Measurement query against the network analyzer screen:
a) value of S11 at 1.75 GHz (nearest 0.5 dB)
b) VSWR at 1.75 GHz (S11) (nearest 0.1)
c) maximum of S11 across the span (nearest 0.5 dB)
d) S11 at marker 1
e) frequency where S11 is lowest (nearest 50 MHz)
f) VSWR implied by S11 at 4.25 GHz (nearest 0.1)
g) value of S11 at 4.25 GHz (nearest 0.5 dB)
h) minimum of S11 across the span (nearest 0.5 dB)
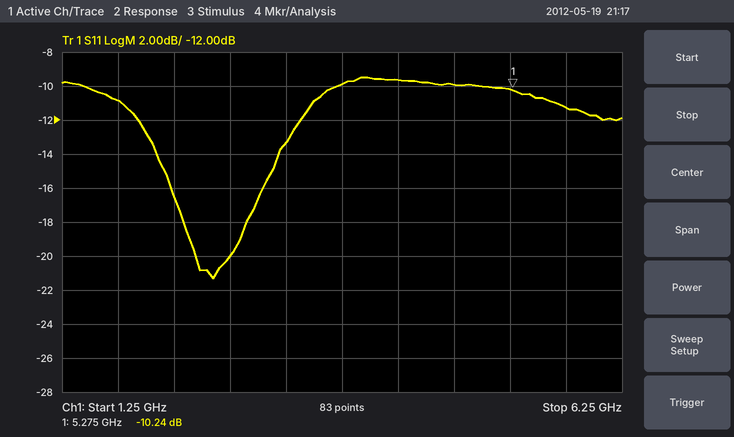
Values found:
-11.0 dB
1.8
-9.5 dB
-10.24 dB
2.60 GHz
2.0
-9.5 dB
-21.5 dB
